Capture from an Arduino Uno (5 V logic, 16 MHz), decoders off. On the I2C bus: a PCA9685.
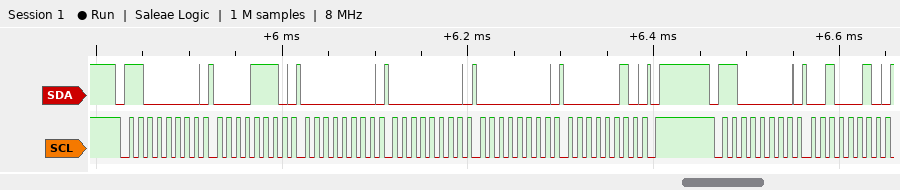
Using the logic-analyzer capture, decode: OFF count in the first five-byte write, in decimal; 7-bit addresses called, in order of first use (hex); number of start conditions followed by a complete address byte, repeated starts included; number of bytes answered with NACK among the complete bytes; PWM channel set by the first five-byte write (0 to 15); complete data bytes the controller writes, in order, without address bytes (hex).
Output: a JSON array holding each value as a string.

["512", "0x60", "2", "0", "2", "0E 00 00 00 02 22"]
